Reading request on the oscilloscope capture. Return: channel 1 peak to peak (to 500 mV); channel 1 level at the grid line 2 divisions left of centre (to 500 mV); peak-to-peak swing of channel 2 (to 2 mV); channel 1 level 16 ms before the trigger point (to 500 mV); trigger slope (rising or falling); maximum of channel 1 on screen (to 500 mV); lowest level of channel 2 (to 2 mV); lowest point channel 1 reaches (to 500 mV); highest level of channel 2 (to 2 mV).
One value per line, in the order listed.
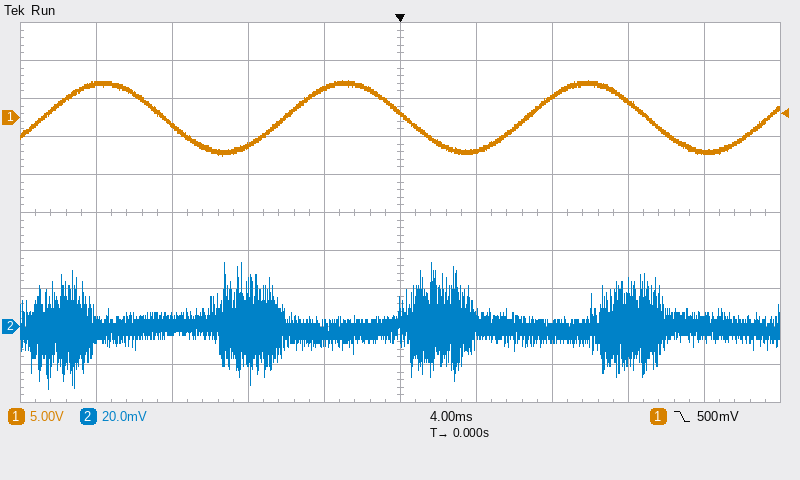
10.0 V
-3.5 V
66 mV
4.5 V
falling
5.0 V
-32 mV
-5.0 V
34 mV
